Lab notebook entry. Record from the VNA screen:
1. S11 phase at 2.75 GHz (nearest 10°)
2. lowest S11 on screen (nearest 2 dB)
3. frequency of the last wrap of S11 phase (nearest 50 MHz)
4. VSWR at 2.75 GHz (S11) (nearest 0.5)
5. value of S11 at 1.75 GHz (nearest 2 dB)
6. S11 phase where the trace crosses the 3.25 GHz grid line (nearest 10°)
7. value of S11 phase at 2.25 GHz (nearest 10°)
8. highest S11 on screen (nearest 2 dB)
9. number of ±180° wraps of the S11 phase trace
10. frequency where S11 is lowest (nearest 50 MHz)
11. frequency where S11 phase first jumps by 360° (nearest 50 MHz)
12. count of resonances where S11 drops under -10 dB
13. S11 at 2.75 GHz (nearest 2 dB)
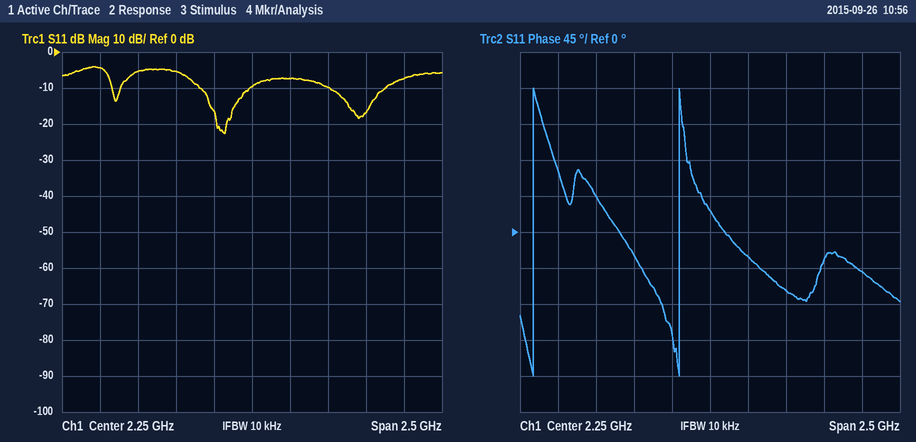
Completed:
-70°
-22 dB
2.05 GHz
2.0
-6 dB
-50°
30°
-4 dB
2
2.05 GHz
1.10 GHz
3
-10 dB
